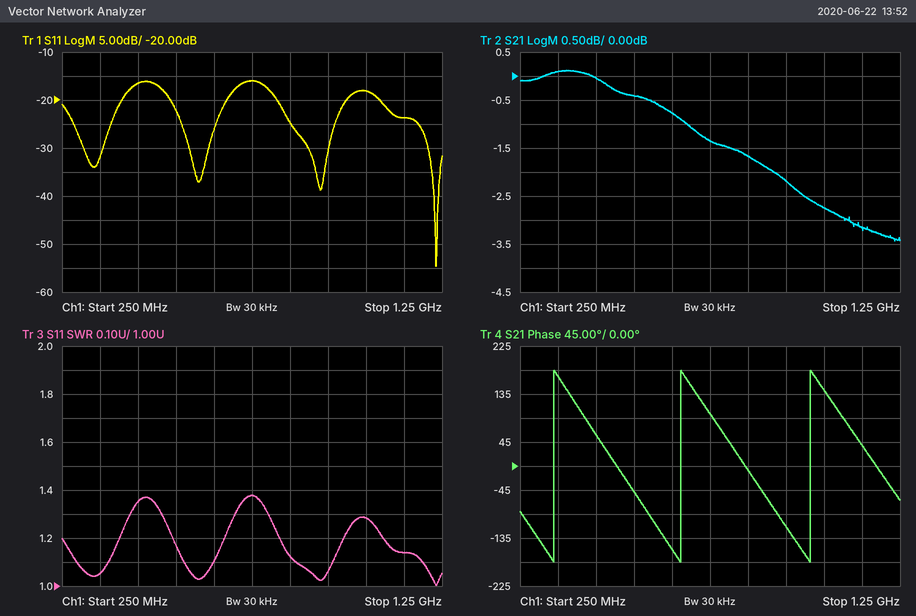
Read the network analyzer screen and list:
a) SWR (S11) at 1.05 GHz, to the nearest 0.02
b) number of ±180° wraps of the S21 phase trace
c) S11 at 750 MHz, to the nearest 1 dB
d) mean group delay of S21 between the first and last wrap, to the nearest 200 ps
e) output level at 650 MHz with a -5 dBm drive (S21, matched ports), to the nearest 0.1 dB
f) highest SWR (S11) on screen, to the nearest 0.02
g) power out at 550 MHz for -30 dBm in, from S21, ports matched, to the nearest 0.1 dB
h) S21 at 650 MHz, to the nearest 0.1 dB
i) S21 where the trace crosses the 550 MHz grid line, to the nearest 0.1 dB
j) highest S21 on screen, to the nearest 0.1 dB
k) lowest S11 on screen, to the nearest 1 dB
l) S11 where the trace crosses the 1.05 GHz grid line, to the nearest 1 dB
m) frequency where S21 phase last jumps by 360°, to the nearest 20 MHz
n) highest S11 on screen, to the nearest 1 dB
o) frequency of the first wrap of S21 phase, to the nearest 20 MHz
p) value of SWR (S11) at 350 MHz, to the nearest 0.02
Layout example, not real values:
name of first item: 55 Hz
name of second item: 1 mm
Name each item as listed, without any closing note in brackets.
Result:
SWR (S11) at 1.05 GHz, to the nearest 0.02: 1.28
number of ±180° wraps of the S21 phase trace: 3
S11 at 750 MHz, to the nearest 1 dB: -16 dB
mean group delay of S21 between the first and last wrap, to the nearest 200 ps: 3.0 ns
output level at 650 MHz with a -5 dBm drive (S21, matched ports), to the nearest 0.1 dB: -5.8 dBm
highest SWR (S11) on screen, to the nearest 0.02: 1.38
power out at 550 MHz for -30 dBm in, from S21, ports matched, to the nearest 0.1 dB: -30.4 dBm
S21 at 650 MHz, to the nearest 0.1 dB: -0.8 dB
S21 where the trace crosses the 550 MHz grid line, to the nearest 0.1 dB: -0.4 dB
highest S21 on screen, to the nearest 0.1 dB: 0.1 dB
lowest S11 on screen, to the nearest 1 dB: -55 dB
S11 where the trace crosses the 1.05 GHz grid line, to the nearest 1 dB: -18 dB
frequency where S21 phase last jumps by 360°, to the nearest 20 MHz: 1.02 GHz
highest S11 on screen, to the nearest 1 dB: -16 dB
frequency of the first wrap of S21 phase, to the nearest 20 MHz: 340 MHz
value of SWR (S11) at 350 MHz, to the nearest 0.02: 1.06
